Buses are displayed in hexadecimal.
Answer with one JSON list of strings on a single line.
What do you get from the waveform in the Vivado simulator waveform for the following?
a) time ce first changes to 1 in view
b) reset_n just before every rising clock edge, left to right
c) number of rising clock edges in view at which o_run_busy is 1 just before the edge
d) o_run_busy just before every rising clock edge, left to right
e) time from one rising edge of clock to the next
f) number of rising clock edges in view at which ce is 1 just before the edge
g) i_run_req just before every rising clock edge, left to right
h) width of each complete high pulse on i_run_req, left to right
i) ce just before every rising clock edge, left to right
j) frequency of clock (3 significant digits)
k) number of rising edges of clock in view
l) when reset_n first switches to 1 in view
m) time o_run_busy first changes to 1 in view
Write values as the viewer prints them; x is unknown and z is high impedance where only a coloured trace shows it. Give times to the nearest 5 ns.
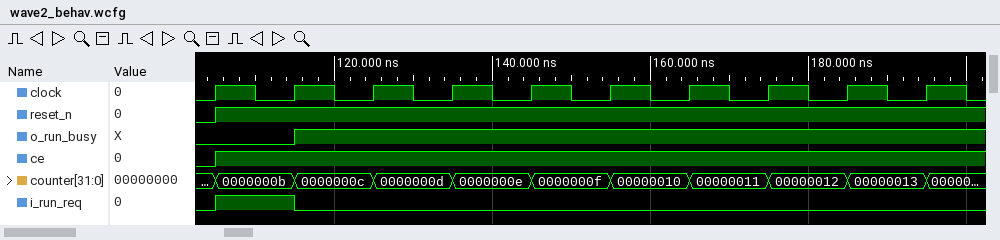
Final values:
["105 ns", "0 1 1 1 1 1 1 1 1 1", "8", "0 0 1 1 1 1 1 1 1 1", "10 ns", "9", "0 1 0 0 0 0 0 0 0 0", "10 ns", "0 1 1 1 1 1 1 1 1 1", "100 MHz", "10", "105 ns", "115 ns"]
